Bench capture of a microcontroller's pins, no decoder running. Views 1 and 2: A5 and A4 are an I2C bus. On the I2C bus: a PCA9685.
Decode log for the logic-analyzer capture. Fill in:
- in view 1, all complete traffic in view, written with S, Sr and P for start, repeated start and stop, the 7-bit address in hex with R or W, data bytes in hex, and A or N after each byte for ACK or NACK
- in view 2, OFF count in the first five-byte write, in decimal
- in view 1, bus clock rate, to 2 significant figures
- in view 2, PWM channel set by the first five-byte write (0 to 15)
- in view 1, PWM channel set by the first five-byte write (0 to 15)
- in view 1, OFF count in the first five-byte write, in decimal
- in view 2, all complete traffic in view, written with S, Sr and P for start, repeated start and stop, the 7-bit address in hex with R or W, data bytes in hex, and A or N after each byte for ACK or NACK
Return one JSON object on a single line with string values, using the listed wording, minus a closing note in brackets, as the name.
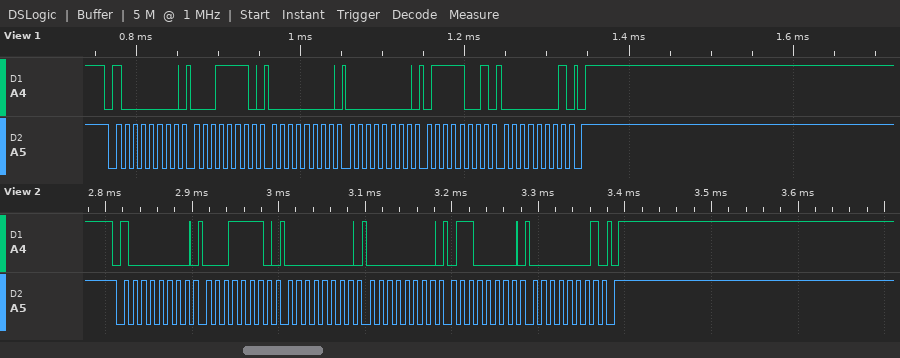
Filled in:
{"in view 1, all complete traffic in view, written with S, Sr and P for start, repeated start and stop, the 7-bit address in hex with R or W, data bytes in hex, and A or N after each byte for ACK or NACK": "S 40W A 1E A 00 A 00 A 79 A 01 A P", "in view 2, OFF count in the first five-byte write, in decimal": "352", "in view 1, bus clock rate, to 2 significant figures": "100 kHz", "in view 2, PWM channel set by the first five-byte write": "6", "in view 1, PWM channel set by the first five-byte write": "6", "in view 1, OFF count in the first five-byte write, in decimal": "377", "in view 2, all complete traffic in view, written with S, Sr and P for start, repeated start and stop, the 7-bit address in hex with R or W, data bytes in hex, and A or N after each byte for ACK or NACK": "S 40W A 1E A 00 A 00 A 60 A 01 A P"}
